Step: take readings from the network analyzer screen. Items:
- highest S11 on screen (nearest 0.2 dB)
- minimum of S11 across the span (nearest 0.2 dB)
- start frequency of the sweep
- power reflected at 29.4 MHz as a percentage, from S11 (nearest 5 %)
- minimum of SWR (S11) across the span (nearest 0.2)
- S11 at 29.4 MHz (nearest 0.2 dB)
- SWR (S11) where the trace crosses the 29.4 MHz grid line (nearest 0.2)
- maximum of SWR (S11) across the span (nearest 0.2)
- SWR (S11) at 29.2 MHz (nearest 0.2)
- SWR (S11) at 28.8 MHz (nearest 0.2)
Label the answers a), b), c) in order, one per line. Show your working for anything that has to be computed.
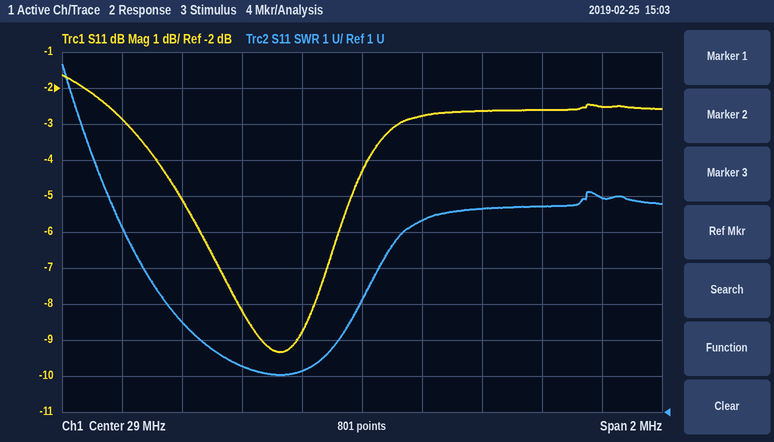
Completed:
a) -1.6 dB
b) -9.4 dB
c) 28 MHz
d) 10^(-2.6/10) ≈ 55 %
e) 2.0
f) -2.6 dB
g) 6.6
h) 10.6
i) 6.4
j) 2.2
